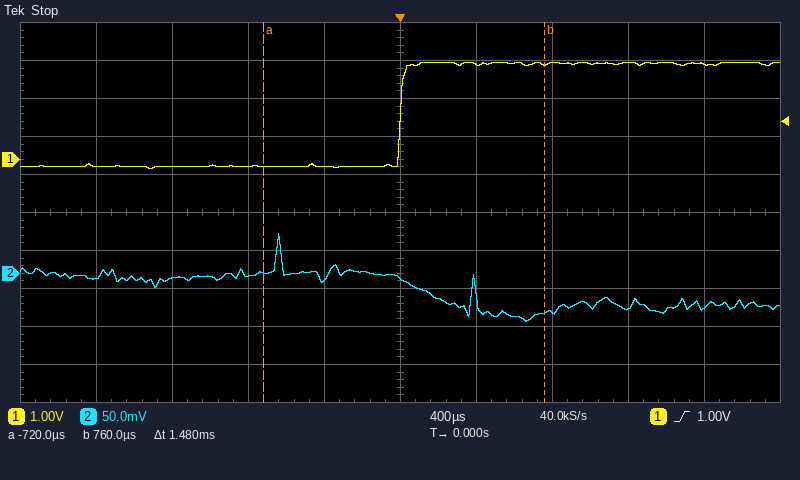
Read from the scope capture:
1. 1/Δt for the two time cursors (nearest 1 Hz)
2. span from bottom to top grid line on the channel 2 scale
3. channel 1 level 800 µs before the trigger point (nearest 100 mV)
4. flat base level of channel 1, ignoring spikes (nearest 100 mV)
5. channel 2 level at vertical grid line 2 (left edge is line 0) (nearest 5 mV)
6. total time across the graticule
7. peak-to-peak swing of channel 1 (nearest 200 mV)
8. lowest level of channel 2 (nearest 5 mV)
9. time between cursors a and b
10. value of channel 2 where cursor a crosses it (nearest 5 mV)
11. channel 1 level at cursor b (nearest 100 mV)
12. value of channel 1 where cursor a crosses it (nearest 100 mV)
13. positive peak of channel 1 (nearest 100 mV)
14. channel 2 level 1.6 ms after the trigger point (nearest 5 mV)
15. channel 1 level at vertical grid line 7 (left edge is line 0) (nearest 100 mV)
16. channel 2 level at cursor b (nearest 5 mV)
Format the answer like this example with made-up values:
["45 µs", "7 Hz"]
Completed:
["676 Hz", "500 mV", "-200 mV", "-200 mV", "-5 mV", "4 ms", "2.8 V", "-65 mV", "1.48 ms", "0 mV", "2.5 V", "-200 mV", "2.5 V", "-45 mV", "2.5 V", "-50 mV"]
